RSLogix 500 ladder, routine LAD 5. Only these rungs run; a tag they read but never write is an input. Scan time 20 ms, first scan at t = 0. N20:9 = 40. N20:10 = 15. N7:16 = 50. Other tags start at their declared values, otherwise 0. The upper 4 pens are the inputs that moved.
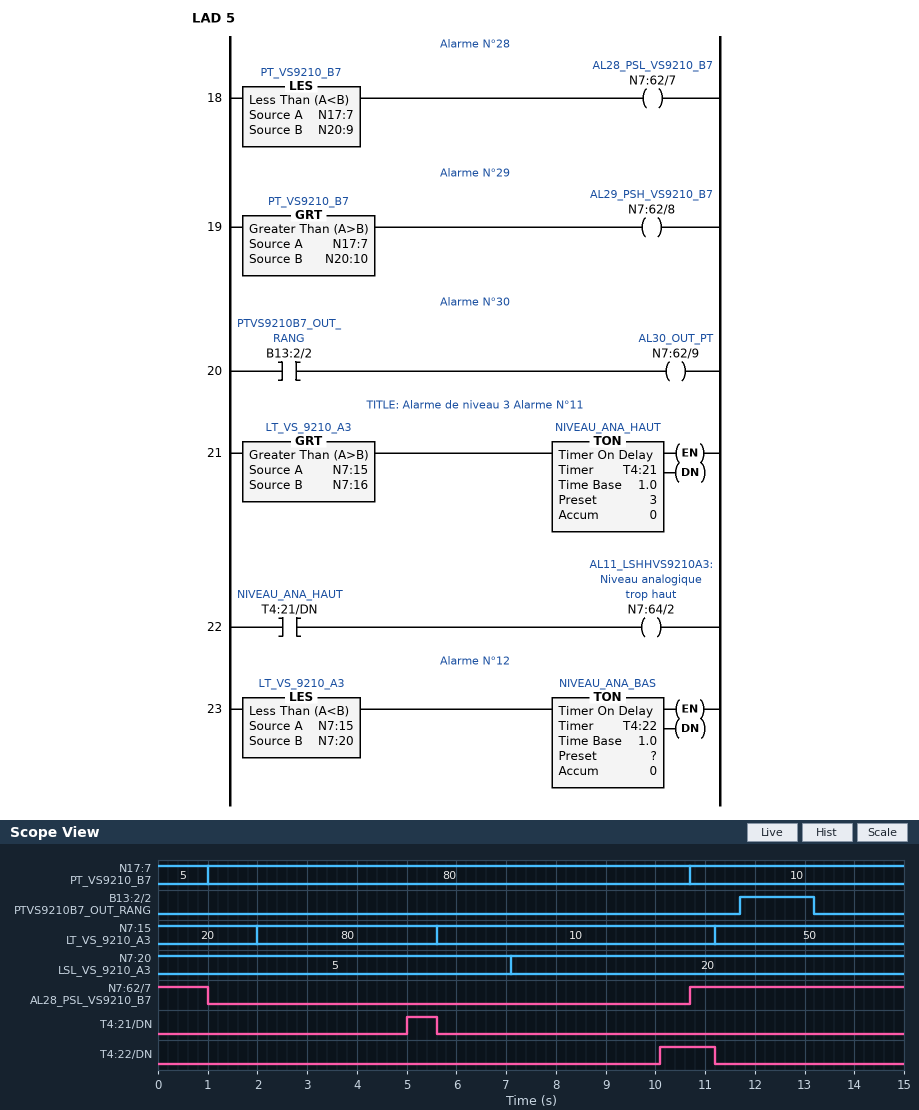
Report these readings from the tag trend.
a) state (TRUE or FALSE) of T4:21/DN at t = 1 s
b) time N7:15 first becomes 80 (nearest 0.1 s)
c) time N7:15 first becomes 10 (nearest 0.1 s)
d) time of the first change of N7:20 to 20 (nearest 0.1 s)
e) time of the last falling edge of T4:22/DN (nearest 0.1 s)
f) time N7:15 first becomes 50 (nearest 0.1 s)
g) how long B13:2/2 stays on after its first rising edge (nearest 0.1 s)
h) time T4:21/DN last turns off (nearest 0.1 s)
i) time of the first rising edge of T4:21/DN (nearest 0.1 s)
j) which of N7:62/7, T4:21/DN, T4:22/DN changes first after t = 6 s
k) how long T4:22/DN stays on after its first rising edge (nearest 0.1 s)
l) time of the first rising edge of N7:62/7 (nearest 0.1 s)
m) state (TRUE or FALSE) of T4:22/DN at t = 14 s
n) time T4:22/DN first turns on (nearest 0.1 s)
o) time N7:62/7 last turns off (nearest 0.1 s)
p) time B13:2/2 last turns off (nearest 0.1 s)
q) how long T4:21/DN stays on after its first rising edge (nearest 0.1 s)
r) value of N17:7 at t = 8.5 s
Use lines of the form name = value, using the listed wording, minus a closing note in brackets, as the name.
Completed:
state (TRUE or FALSE) of T4:21/DN at t = 1 s = FALSE
time N7:15 first becomes 80 = 2.0 s
time N7:15 first becomes 10 = 5.6 s
time of the first change of N7:20 to 20 = 7.1 s
time of the last falling edge of T4:22/DN = 11.2 s
time N7:15 first becomes 50 = 11.2 s
how long B13:2/2 stays on after its first rising edge = 1.5 s
time T4:21/DN last turns off = 5.6 s
time of the first rising edge of T4:21/DN = 5.0 s
which of N7:62/7, T4:21/DN, T4:22/DN changes first after t = 6 s = T4:22/DN
how long T4:22/DN stays on after its first rising edge = 1.1 s
time of the first rising edge of N7:62/7 = 10.7 s
state (TRUE or FALSE) of T4:22/DN at t = 14 s = FALSE
time T4:22/DN first turns on = 10.1 s
time N7:62/7 last turns off = 1.0 s
time B13:2/2 last turns off = 13.2 s
how long T4:21/DN stays on after its first rising edge = 0.6 s
value of N17:7 at t = 8.5 s = 80
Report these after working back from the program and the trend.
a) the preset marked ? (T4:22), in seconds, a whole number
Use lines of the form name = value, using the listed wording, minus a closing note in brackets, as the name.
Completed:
the preset marked ? (T4:22), in seconds, a whole number = 3 s
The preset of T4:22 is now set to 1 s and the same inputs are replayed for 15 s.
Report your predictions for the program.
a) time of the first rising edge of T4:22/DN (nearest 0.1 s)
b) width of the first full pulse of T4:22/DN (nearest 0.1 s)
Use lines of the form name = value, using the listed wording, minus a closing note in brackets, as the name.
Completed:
time of the first rising edge of T4:22/DN = 8.1 s
width of the first full pulse of T4:22/DN = 3.1 s
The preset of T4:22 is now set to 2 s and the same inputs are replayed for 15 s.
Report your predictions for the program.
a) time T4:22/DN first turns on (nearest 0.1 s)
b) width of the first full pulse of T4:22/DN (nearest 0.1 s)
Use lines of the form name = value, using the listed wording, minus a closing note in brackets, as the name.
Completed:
time T4:22/DN first turns on = 9.1 s
width of the first full pulse of T4:22/DN = 2.1 s
